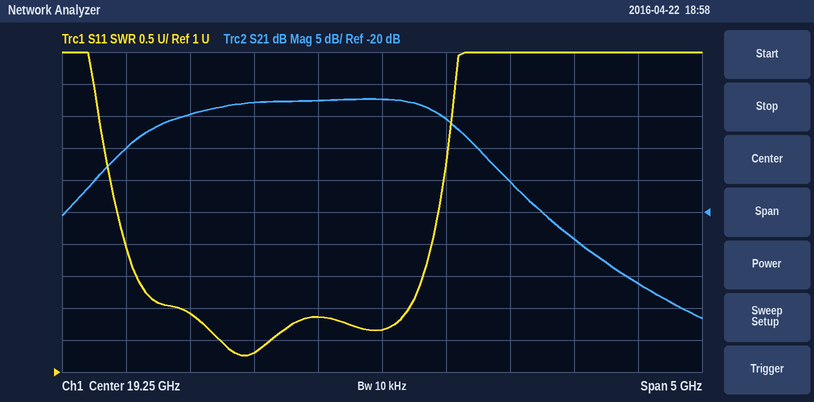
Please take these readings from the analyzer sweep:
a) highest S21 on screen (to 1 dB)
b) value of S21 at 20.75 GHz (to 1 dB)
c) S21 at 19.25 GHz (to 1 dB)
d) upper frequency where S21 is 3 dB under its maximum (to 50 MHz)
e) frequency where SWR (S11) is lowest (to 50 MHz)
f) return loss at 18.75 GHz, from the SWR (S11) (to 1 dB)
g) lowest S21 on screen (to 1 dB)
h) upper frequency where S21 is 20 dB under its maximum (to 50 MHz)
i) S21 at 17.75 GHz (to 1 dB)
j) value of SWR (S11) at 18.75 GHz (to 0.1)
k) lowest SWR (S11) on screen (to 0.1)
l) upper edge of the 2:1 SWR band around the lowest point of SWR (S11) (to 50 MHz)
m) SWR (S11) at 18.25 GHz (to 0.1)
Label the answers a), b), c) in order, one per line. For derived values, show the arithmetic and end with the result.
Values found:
a) -2 dB
b) -24 dB
c) -2 dB
d) 19.75 GHz
e) 18.15 GHz
f) −20 log10((1.9 − 1)/(1.9 + 1)) ≈ 10 dB
g) -37 dB
h) 20.65 GHz
i) -5 dB
j) 1.9
k) 1.3
l) 19.45 GHz
m) 1.3
